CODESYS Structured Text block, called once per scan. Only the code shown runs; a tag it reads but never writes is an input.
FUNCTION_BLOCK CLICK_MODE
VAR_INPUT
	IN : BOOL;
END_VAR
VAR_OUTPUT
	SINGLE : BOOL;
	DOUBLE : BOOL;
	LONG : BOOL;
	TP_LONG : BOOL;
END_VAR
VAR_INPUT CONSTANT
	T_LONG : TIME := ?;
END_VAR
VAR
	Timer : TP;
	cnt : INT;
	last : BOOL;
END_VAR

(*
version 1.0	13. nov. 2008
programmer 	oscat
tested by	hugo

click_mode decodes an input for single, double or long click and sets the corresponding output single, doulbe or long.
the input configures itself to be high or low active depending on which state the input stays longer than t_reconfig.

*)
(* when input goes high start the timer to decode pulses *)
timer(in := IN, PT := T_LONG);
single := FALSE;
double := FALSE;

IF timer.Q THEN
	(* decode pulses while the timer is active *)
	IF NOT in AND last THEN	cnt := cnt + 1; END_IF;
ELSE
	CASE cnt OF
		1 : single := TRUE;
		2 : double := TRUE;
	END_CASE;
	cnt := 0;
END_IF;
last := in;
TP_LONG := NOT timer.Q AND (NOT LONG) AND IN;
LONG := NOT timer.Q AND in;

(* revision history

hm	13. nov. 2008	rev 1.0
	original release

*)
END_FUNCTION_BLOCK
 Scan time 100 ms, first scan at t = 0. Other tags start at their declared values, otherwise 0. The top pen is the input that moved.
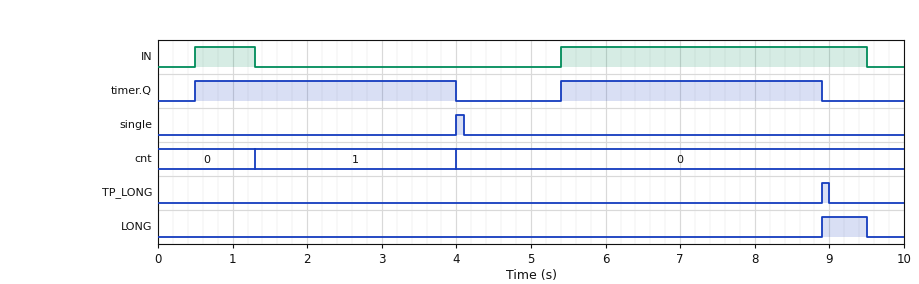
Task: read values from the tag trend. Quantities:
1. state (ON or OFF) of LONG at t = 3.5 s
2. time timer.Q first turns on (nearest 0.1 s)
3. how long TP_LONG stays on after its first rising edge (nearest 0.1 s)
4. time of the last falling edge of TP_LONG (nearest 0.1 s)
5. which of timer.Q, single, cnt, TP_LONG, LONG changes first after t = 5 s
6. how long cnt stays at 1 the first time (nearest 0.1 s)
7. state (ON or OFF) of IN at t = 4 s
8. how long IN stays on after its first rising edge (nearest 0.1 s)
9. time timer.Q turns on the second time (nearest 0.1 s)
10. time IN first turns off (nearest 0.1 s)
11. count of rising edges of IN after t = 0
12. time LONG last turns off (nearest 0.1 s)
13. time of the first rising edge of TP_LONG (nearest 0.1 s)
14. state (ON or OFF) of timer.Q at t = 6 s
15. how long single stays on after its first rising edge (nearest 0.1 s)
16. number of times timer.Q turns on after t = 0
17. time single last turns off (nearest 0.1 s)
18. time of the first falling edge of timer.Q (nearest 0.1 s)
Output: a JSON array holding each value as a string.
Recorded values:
["OFF", "0.5 s", "0.1 s", "9.0 s", "timer.Q", "2.7 s", "OFF", "0.8 s", "5.4 s", "1.3 s", "2", "9.5 s", "8.9 s", "ON", "0.1 s", "2", "4.1 s", "4.0 s"]
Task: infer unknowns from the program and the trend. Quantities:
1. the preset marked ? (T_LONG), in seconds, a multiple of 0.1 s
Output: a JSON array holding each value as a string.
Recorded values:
["3.5 s"]
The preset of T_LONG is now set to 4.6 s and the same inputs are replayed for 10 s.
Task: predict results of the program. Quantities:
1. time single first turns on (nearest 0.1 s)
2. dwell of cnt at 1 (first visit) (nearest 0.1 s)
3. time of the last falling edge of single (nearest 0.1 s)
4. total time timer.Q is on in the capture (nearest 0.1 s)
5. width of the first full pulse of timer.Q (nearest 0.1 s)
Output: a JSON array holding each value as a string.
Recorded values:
["5.1 s", "3.8 s", "5.2 s", "9.2 s", "4.6 s"]
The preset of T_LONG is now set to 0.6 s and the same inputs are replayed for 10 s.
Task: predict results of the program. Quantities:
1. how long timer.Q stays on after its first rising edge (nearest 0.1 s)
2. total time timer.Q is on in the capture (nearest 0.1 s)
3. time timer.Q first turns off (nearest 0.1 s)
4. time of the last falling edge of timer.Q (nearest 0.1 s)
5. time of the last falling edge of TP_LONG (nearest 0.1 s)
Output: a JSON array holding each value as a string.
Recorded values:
["0.6 s", "1.2 s", "1.1 s", "6.0 s", "6.1 s"]
